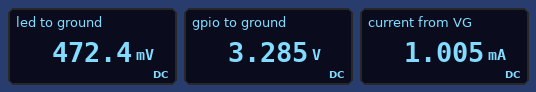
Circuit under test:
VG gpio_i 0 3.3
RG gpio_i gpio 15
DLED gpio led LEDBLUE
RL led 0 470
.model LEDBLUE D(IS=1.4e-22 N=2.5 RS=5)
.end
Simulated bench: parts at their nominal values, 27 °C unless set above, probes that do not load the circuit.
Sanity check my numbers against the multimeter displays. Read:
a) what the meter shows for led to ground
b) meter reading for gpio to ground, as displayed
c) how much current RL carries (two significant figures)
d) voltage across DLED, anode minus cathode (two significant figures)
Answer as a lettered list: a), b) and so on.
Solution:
a) 472.4 mV
b) 3.285 V
c) 1.0 mA
d) 2.8 V
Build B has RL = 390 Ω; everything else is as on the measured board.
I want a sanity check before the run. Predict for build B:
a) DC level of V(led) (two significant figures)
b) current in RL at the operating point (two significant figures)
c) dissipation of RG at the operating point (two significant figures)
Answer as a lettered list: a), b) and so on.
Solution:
a) 460 mV
b) 1.2 mA
c) 21 µW
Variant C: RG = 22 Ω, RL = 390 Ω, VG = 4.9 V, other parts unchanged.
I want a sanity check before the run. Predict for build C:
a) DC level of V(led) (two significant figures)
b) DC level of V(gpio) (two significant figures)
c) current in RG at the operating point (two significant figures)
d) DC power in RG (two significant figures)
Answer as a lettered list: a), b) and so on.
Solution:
a) 1.9 V
b) 4.8 V
c) 4.8 mA
d) 500 µW
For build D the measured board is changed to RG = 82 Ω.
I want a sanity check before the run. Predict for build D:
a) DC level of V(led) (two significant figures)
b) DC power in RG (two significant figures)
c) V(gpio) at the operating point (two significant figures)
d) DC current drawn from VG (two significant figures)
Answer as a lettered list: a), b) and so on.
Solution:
a) 420 mV
b) 66 µW
c) 3.2 V
d) 900 µA
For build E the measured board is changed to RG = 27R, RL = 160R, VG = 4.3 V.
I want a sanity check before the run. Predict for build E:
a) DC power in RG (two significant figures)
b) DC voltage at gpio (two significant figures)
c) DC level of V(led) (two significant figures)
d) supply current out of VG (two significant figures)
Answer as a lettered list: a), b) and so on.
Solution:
a) 1.4 mW
b) 4.1 V
c) 1.1 V
d) 7.1 mA
